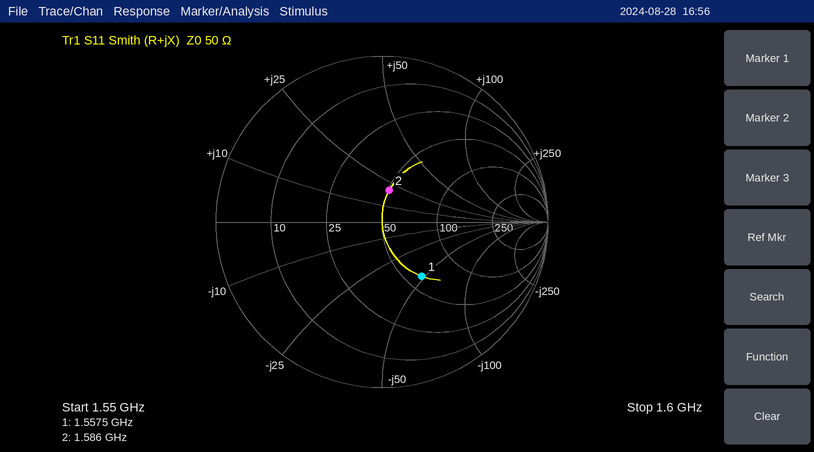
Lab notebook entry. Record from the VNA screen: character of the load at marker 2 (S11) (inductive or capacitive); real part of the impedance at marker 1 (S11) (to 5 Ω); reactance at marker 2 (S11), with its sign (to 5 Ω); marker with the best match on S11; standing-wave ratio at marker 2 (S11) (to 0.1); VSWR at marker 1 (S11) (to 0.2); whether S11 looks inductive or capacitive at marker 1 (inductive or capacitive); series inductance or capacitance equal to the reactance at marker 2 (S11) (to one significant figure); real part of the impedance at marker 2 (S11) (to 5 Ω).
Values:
inductive
60 Ω
+20 Ω
marker 2
1.5
2.4
capacitive
2 nH
50 Ω
